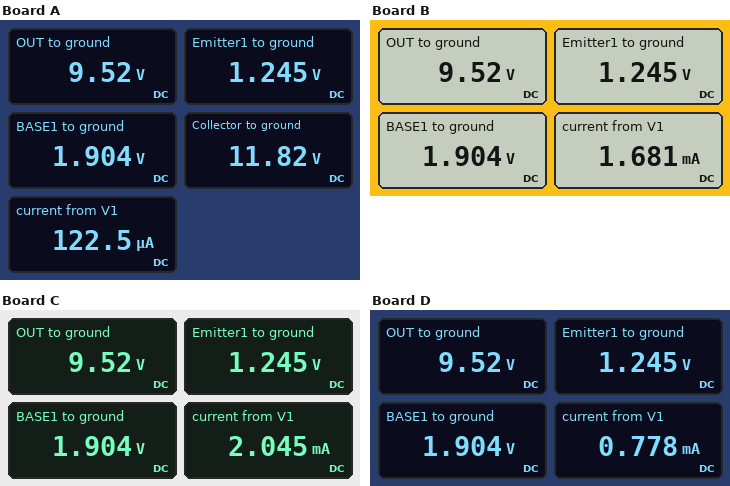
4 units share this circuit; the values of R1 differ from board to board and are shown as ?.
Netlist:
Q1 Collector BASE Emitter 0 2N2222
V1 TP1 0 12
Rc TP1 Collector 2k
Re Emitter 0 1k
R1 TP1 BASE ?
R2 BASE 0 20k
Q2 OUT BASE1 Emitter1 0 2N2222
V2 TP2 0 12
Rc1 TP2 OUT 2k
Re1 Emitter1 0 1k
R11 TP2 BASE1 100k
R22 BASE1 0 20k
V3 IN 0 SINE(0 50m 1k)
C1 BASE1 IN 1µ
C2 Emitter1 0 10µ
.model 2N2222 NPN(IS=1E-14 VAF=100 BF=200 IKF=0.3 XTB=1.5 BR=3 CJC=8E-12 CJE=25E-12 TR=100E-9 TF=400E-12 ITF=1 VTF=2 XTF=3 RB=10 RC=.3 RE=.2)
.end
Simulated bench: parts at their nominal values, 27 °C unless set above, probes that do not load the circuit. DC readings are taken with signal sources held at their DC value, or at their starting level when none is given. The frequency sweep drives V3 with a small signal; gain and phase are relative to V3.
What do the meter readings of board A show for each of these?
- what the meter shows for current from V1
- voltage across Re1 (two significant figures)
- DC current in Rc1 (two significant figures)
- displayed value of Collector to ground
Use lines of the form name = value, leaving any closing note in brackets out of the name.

what the meter shows for current from V1 = 122.5 µA
voltage across Re1 = 1.2 V
DC current in Rc1 = 1.2 mA
displayed value of Collector to ground = 11.82 V
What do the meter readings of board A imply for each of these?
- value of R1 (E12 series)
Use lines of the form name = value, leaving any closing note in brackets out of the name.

value of R1 = 330 kΩ
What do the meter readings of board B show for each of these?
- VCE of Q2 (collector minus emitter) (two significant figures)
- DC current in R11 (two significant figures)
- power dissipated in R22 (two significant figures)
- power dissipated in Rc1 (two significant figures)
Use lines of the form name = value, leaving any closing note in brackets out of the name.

VCE of Q2 (collector minus emitter) = 8.3 V
DC current in R11 = 100 µA
power dissipated in R22 = 180 µW
power dissipated in Rc1 = 3.1 mW
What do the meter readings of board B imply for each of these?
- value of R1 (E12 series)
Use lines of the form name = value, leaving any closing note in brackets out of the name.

value of R1 = 82 kΩ
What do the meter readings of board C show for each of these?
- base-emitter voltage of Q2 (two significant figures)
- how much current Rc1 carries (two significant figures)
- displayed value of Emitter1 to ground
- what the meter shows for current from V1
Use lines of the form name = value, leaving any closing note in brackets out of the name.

base-emitter voltage of Q2 = 660 mV
how much current Rc1 carries = 1.2 mA
displayed value of Emitter1 to ground = 1.245 V
what the meter shows for current from V1 = 2.045 mA
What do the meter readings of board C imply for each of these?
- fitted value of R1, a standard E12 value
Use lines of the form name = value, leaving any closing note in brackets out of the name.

fitted value of R1, a standard E12 value = 68 kΩ
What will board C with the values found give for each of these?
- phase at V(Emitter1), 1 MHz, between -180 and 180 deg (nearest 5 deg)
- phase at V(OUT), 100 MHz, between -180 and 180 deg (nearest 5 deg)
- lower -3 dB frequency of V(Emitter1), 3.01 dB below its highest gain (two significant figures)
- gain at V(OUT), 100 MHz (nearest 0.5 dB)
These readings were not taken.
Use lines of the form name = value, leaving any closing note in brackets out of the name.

phase at V(Emitter1), 1 MHz, between -180 and 180 deg = -90 deg
phase at V(OUT), 100 MHz, between -180 and 180 deg = 80 deg
lower -3 dB frequency of V(Emitter1), 3.01 dB below its highest gain = 9.6 Hz
gain at V(OUT), 100 MHz = 22.5 dB
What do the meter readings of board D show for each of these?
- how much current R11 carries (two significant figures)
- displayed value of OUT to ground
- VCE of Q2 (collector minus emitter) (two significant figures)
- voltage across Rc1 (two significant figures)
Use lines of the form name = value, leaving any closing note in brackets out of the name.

how much current R11 carries = 100 µA
displayed value of OUT to ground = 9.52 V
VCE of Q2 (collector minus emitter) = 8.3 V
voltage across Rc1 = 2.5 V
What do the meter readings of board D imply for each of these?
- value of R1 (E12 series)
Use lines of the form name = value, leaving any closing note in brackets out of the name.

value of R1 = 150 kΩ
